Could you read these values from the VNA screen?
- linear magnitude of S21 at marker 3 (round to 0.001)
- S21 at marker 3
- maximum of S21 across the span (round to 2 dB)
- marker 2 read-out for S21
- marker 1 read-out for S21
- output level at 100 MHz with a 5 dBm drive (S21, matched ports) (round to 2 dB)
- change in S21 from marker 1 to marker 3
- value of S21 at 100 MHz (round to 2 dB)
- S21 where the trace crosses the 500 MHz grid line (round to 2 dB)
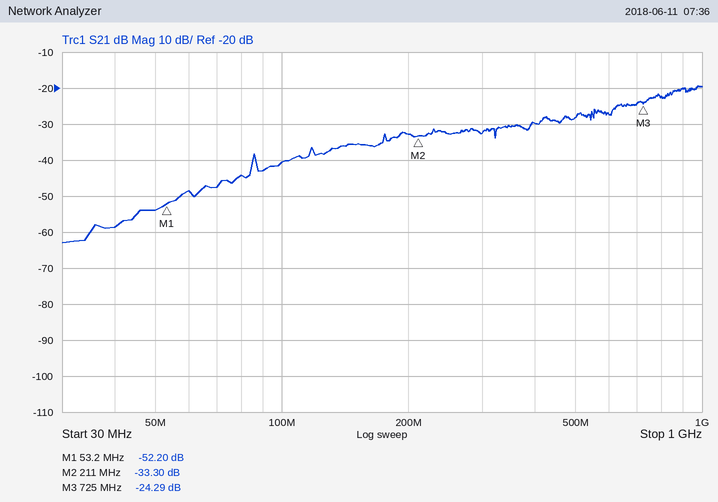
0.061
-24.29 dB
-20 dB
-33.30 dB
-52.20 dB
-36 dBm
27.91 dB
-40 dB
-28 dB
